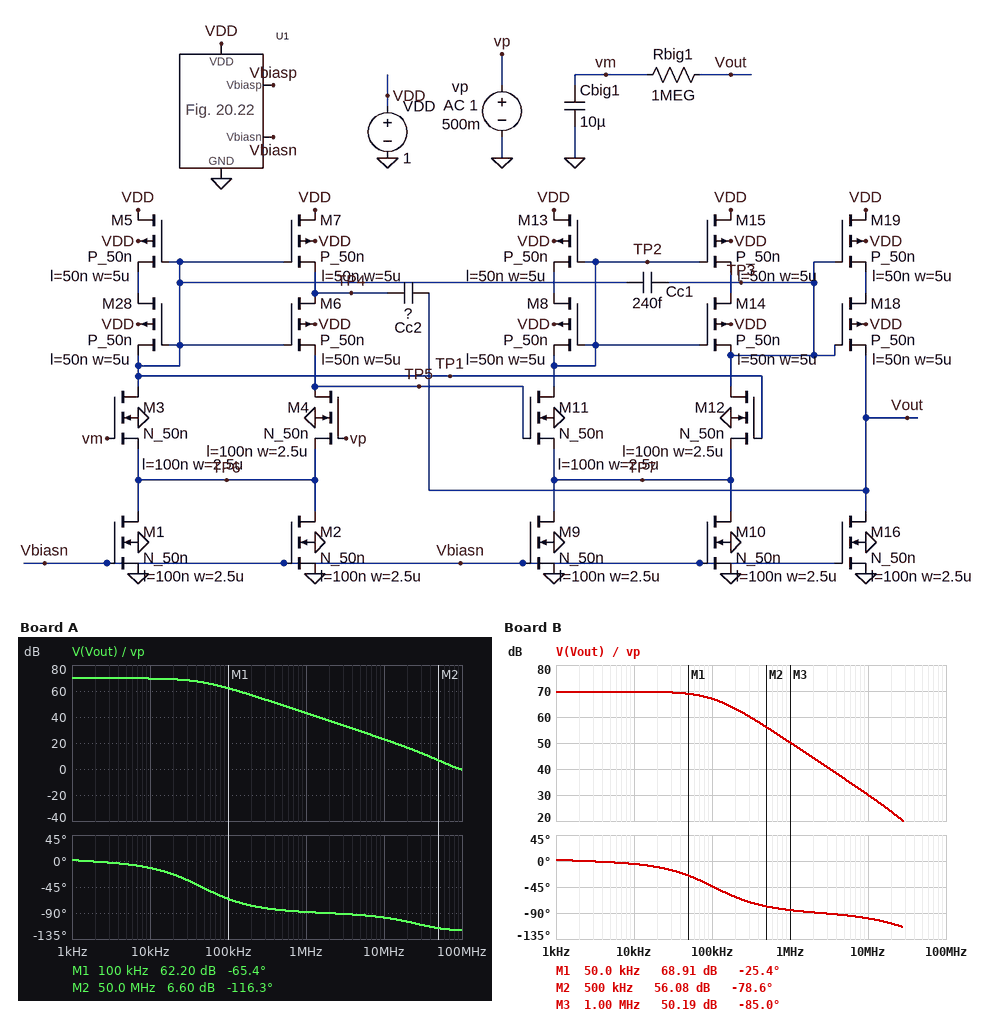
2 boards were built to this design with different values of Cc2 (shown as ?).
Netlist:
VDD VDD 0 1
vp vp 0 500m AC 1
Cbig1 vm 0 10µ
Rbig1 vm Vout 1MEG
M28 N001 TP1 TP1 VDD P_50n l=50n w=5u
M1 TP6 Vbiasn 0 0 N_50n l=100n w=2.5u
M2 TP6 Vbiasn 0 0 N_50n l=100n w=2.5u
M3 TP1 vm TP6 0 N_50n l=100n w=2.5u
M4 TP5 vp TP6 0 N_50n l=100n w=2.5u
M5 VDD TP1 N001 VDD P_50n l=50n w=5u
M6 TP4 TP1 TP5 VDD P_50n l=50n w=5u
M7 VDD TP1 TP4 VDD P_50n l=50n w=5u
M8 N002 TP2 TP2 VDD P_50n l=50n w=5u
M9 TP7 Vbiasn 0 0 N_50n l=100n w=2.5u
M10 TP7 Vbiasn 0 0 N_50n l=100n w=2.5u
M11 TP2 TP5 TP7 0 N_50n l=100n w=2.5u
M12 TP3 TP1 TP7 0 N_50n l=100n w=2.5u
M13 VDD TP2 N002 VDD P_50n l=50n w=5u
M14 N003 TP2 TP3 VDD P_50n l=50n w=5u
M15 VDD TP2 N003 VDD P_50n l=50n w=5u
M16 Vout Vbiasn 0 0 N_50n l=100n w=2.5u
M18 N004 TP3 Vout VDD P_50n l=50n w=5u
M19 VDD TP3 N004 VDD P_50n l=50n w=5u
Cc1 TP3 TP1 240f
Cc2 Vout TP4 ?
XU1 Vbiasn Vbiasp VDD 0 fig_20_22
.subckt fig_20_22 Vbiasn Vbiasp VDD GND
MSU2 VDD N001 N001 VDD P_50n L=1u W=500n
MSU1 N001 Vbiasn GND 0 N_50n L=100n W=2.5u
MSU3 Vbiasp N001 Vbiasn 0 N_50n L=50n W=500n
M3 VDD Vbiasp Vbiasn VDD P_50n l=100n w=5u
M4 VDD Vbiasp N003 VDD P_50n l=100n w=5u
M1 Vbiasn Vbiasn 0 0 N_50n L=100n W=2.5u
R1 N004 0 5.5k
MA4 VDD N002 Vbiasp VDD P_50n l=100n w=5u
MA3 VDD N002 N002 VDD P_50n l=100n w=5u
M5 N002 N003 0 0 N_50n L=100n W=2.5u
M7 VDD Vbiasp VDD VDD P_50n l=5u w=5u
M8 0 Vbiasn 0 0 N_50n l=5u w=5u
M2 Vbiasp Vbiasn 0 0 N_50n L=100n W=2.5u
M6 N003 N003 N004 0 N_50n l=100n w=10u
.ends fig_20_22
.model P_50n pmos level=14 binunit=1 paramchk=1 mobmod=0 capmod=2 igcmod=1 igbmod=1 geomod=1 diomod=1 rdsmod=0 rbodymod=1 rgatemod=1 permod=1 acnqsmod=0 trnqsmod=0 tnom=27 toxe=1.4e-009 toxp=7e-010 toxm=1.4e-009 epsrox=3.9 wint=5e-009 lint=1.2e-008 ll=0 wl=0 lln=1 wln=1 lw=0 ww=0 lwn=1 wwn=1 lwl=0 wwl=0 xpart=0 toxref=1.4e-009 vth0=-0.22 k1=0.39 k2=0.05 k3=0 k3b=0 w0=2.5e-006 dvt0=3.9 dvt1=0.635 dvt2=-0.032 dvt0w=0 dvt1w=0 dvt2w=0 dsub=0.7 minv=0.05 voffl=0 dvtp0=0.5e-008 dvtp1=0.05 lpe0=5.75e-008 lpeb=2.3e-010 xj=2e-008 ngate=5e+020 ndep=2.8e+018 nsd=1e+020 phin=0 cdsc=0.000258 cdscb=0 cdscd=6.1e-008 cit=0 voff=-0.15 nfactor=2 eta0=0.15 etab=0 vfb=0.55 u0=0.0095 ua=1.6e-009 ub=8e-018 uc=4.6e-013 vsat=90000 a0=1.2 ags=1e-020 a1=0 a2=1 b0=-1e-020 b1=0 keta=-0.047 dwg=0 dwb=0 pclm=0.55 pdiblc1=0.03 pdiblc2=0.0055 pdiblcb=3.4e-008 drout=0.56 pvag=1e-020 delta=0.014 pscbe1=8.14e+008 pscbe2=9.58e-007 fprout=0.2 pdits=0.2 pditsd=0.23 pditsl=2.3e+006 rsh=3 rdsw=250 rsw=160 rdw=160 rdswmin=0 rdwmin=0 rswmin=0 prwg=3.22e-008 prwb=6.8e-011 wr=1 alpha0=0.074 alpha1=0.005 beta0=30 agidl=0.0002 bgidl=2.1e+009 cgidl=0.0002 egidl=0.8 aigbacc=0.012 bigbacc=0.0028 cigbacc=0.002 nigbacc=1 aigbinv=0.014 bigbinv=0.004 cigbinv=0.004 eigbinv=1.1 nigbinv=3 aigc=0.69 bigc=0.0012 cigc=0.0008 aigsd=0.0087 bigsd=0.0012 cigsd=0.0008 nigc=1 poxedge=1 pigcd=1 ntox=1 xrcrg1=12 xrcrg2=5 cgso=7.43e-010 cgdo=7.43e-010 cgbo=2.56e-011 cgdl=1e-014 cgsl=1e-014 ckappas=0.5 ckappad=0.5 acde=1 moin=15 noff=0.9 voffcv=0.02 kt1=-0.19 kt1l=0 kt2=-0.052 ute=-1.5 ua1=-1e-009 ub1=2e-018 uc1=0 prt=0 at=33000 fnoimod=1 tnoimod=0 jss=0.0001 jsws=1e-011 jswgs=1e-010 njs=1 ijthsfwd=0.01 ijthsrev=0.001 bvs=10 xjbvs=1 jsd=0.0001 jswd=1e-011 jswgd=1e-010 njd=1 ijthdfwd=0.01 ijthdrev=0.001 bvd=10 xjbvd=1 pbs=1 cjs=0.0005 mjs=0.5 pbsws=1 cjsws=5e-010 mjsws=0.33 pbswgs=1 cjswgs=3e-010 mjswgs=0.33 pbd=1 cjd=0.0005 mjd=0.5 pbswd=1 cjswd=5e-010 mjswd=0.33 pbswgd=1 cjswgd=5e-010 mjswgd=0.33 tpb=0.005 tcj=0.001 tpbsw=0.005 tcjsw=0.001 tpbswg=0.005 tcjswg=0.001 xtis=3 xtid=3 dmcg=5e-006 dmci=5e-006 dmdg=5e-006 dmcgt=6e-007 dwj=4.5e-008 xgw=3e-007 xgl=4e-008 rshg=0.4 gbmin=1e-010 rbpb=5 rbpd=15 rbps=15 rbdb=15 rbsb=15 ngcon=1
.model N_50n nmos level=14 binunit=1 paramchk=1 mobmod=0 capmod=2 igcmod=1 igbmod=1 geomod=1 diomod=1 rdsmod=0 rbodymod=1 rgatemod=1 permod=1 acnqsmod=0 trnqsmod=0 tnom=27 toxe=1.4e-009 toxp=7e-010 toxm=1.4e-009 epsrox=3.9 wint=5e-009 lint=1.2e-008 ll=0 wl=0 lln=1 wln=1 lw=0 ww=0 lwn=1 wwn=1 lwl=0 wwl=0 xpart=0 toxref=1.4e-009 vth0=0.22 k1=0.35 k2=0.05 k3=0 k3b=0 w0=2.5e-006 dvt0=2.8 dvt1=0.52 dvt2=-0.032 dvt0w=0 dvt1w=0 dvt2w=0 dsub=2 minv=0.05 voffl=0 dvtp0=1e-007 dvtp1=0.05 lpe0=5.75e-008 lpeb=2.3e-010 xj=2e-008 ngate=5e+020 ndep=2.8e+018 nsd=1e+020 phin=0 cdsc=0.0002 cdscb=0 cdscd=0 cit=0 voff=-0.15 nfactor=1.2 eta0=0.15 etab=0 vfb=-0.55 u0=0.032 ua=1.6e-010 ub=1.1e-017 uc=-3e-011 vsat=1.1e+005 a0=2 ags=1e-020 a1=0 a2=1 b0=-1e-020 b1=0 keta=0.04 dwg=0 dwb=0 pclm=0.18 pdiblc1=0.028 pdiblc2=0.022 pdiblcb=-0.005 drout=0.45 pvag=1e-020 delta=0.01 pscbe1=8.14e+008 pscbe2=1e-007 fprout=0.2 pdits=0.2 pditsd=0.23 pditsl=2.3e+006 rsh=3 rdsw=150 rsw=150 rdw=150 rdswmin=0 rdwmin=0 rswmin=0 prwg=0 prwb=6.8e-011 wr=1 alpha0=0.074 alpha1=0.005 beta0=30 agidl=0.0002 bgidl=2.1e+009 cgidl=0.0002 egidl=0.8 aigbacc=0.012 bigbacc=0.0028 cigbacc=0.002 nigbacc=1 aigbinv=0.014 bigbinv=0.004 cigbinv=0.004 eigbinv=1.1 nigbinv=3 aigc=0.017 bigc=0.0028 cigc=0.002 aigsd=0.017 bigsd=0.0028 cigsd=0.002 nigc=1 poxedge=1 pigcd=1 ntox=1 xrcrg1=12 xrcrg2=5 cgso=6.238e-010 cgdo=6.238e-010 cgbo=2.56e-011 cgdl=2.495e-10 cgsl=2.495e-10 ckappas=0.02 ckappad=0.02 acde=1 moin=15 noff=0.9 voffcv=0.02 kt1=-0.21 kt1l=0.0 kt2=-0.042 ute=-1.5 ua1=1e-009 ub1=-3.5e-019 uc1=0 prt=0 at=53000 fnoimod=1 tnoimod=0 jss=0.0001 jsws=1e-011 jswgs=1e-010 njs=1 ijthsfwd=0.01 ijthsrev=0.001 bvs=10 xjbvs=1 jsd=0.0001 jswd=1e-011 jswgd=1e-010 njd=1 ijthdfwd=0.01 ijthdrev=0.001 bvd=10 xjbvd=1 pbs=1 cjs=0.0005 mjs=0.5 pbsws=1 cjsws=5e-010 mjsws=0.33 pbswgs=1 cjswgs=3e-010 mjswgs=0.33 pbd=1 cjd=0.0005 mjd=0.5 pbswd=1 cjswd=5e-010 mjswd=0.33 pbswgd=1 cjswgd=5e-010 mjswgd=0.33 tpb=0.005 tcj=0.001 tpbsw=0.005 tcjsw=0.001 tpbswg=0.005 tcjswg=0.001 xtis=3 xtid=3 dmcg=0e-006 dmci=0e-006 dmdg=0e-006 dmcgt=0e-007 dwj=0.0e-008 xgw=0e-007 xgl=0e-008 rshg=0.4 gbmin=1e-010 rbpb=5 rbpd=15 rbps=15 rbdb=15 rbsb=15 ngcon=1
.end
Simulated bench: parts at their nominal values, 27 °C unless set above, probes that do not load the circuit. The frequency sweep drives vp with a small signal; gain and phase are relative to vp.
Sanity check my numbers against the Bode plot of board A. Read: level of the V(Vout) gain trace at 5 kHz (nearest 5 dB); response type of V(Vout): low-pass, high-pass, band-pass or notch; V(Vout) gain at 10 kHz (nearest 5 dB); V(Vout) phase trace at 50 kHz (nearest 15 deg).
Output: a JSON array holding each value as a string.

["70 dB", "low-pass", "70 dB", "-45 deg"]
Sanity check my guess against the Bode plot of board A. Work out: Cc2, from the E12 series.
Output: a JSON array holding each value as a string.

["270 fF"]
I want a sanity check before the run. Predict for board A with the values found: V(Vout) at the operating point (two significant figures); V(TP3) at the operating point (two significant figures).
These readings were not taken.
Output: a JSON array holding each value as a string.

["500 mV", "670 mV"]
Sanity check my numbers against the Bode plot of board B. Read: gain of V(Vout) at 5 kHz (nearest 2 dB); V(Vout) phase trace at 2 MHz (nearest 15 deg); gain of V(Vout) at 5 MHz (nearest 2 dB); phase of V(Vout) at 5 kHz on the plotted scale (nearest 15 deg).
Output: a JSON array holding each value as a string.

["70 dB", "-90 deg", "36 dB", "0 deg"]
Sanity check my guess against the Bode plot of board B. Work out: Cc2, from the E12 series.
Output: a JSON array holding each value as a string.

["100 fF"]
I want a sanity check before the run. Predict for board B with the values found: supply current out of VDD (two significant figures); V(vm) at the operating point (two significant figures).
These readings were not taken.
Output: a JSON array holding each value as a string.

["96 µA", "500 mV"]
